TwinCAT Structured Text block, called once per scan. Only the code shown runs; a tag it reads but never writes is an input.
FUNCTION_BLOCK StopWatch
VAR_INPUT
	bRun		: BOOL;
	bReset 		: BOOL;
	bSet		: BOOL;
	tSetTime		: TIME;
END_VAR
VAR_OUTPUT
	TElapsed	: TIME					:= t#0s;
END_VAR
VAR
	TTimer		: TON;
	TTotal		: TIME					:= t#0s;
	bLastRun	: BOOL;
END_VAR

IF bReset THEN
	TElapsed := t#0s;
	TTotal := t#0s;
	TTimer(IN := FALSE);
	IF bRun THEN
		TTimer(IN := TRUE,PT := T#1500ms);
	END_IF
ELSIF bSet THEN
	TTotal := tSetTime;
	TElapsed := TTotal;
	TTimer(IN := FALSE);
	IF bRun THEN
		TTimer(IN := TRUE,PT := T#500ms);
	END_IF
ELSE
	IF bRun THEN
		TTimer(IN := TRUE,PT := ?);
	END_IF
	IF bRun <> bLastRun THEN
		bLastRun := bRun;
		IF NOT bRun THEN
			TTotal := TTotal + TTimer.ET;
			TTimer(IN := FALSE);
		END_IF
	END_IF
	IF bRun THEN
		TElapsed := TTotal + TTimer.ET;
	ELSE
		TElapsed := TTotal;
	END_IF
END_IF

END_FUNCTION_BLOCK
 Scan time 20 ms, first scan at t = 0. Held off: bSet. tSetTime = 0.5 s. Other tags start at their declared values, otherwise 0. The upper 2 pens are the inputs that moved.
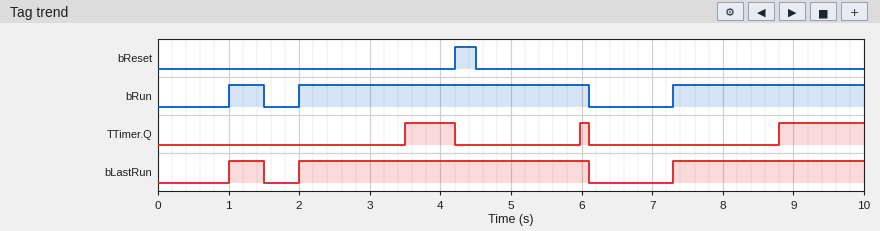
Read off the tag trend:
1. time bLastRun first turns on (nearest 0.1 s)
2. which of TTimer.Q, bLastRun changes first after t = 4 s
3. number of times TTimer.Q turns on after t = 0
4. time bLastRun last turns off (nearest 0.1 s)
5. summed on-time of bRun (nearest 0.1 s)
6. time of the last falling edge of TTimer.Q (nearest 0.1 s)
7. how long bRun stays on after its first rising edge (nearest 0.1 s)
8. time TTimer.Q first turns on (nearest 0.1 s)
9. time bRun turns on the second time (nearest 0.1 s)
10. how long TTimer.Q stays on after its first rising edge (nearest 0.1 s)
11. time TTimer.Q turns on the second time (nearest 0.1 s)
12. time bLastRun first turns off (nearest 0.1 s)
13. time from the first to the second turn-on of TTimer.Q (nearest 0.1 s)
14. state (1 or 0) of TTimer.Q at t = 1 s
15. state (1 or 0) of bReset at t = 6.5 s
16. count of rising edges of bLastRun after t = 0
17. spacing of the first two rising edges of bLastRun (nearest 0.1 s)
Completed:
1.0 s
TTimer.Q
3
6.1 s
7.3 s
6.1 s
0.5 s
3.5 s
2.0 s
0.7 s
6.0 s
1.5 s
2.5 s
0
0
3
1.0 s
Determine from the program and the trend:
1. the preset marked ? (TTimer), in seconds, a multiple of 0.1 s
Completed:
1.5 s
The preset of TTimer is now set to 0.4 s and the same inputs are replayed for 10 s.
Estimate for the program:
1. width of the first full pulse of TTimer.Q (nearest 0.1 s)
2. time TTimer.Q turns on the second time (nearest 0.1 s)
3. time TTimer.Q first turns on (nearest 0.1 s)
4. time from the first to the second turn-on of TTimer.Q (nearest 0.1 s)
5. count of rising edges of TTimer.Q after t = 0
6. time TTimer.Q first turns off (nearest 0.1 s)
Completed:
0.1 s
2.4 s
1.4 s
1.0 s
4
1.5 s
